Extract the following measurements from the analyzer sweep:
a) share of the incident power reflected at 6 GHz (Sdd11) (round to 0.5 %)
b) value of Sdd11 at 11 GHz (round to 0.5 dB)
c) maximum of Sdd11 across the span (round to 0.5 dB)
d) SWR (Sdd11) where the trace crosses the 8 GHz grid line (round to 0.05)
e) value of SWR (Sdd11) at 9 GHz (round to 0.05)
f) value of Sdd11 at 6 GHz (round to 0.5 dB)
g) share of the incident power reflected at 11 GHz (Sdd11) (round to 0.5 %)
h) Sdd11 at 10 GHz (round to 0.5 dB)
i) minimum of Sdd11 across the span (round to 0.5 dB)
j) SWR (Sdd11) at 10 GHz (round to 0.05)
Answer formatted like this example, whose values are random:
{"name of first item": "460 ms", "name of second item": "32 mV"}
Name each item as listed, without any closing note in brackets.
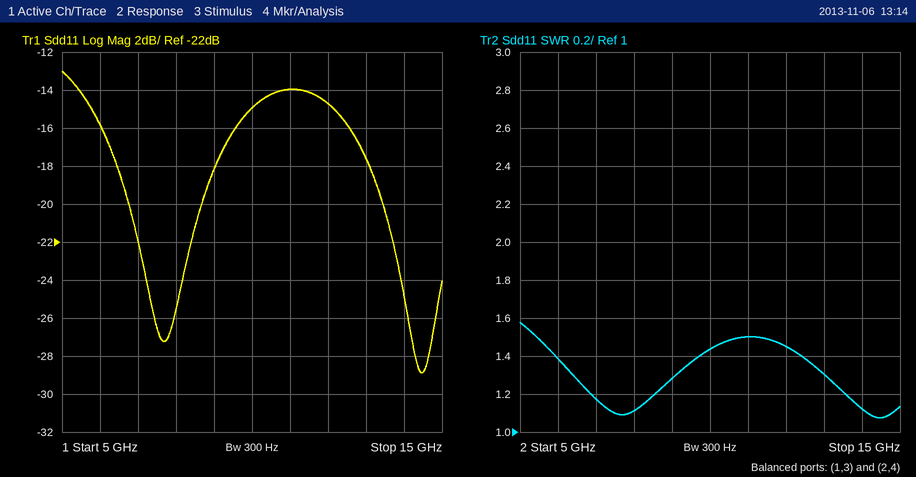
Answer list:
{"share of the incident power reflected at 6 GHz (Sdd11)": "2.5 %", "value of Sdd11 at 11 GHz": "-14.0 dB", "maximum of Sdd11 across the span": "-13.0 dB", "SWR (Sdd11) where the trace crosses the 8 GHz grid line": "1.10", "value of SWR (Sdd11) at 9 GHz": "1.30", "value of Sdd11 at 6 GHz": "-16.0 dB", "share of the incident power reflected at 11 GHz (Sdd11)": "4.0 %", "Sdd11 at 10 GHz": "-15.0 dB", "minimum of Sdd11 across the span": "-29.0 dB", "SWR (Sdd11) at 10 GHz": "1.45"}
